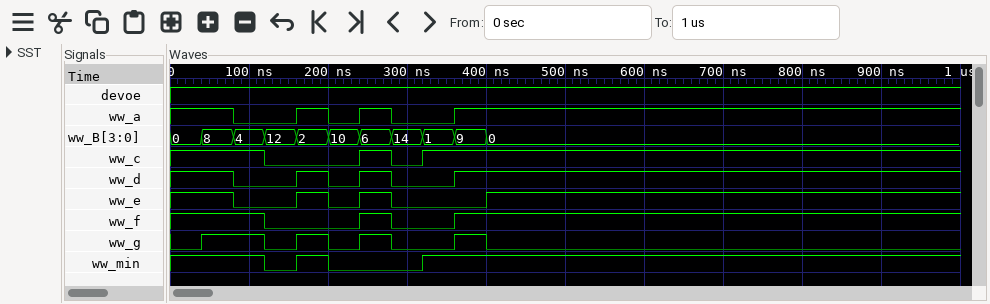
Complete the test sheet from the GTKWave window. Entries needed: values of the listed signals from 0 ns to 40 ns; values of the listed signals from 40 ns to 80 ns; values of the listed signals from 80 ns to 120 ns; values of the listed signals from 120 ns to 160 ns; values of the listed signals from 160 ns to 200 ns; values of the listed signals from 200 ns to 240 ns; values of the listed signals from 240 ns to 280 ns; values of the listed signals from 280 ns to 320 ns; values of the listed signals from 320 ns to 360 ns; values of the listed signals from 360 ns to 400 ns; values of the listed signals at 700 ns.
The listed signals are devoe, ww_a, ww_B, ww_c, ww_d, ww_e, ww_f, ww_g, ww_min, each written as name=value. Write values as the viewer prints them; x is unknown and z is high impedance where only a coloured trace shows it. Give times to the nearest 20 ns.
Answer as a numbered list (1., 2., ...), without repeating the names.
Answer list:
1. devoe=1, ww_a=1, ww_B=0, ww_c=1, ww_d=1, ww_e=1, ww_f=1, ww_g=0, ww_min=1
2. devoe=1, ww_a=1, ww_B=8, ww_c=1, ww_d=1, ww_e=1, ww_f=1, ww_g=1, ww_min=1
3. devoe=1, ww_a=0, ww_B=4, ww_c=1, ww_d=0, ww_e=0, ww_f=1, ww_g=1, ww_min=1
4. devoe=1, ww_a=0, ww_B=12, ww_c=0, ww_d=0, ww_e=0, ww_f=0, ww_g=0, ww_min=0
5. devoe=1, ww_a=1, ww_B=2, ww_c=0, ww_d=1, ww_e=1, ww_f=0, ww_g=1, ww_min=1
6. devoe=1, ww_a=0, ww_B=10, ww_c=0, ww_d=0, ww_e=0, ww_f=0, ww_g=0, ww_min=0
7. devoe=1, ww_a=1, ww_B=6, ww_c=1, ww_d=1, ww_e=1, ww_f=1, ww_g=1, ww_min=0
8. devoe=1, ww_a=0, ww_B=14, ww_c=0, ww_d=0, ww_e=0, ww_f=0, ww_g=0, ww_min=0
9. devoe=1, ww_a=0, ww_B=1, ww_c=1, ww_d=0, ww_e=0, ww_f=0, ww_g=0, ww_min=1
10. devoe=1, ww_a=1, ww_B=9, ww_c=1, ww_d=1, ww_e=0, ww_f=1, ww_g=1, ww_min=1
11. devoe=1, ww_a=1, ww_B=0, ww_c=1, ww_d=1, ww_e=1, ww_f=1, ww_g=0, ww_min=1
